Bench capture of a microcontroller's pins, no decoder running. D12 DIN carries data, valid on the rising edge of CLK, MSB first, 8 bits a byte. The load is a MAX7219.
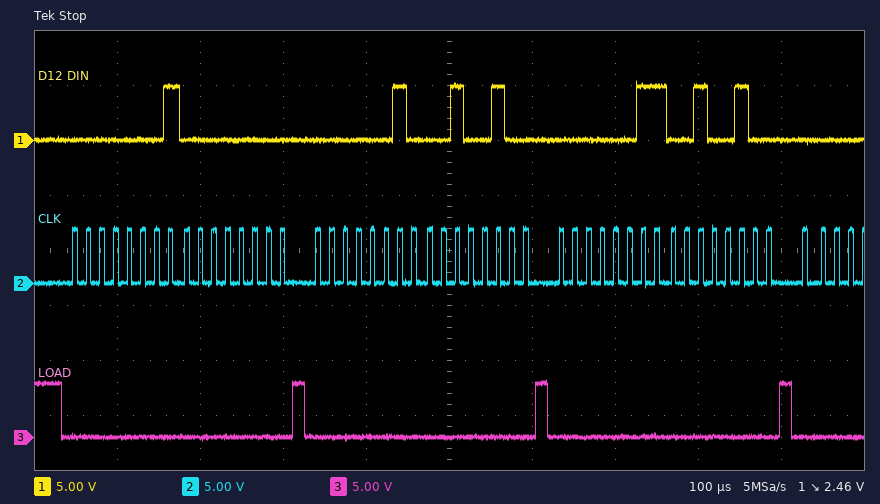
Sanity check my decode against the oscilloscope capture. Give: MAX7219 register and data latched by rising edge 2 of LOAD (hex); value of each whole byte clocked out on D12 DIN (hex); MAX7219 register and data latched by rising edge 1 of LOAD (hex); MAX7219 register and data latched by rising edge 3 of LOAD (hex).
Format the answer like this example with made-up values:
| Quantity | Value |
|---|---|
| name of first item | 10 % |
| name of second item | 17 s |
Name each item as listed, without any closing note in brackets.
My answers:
| Quantity | Value |
|---|---|
| MAX7219 register and data latched by rising edge 2 of LOAD | register 0x2, data 0x24 |
| value of each whole byte clocked out on D12 DIN | 01 00 02 24 03 24 |
| MAX7219 register and data latched by rising edge 1 of LOAD | register 0x1, data 0x00 |
| MAX7219 register and data latched by rising edge 3 of LOAD | register 0x3, data 0x24 |
